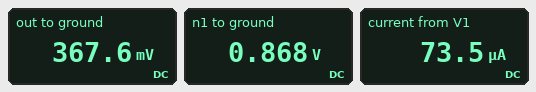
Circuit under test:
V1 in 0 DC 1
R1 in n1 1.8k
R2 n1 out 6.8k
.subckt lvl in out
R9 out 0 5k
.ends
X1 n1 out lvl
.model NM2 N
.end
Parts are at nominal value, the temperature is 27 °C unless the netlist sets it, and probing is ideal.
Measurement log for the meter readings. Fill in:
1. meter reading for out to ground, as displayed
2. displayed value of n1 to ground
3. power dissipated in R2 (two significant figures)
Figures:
367.6 mV
0.868 V
37 µW
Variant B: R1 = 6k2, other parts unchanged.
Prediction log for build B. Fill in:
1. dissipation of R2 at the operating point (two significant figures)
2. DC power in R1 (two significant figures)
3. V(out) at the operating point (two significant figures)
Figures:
21 µW
19 µW
280 mV
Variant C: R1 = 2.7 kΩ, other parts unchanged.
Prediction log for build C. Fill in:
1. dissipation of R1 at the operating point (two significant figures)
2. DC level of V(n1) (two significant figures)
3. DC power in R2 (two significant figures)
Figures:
13 µW
810 mV
32 µW
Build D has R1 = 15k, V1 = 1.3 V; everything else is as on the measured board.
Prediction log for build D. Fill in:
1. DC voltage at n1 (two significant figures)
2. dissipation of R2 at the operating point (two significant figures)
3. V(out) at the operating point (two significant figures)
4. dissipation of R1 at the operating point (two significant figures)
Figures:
570 mV
16 µW
240 mV
35 µW
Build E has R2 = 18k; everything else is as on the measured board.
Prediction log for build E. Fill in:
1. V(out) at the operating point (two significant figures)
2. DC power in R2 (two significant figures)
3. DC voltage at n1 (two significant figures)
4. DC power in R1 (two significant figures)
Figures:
200 mV
29 µW
930 mV
2.9 µW
